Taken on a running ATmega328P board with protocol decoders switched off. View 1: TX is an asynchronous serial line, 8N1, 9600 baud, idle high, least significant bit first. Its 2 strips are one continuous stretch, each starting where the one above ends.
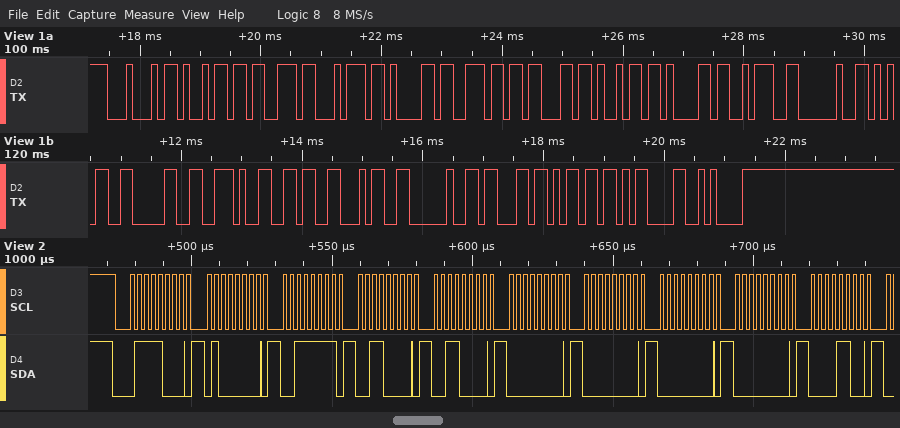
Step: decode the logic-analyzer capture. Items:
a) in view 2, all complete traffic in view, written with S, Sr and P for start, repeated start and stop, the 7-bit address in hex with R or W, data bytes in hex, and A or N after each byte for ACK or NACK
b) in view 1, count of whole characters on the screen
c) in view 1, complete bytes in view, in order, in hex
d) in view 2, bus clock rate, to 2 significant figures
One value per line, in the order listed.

S 3CW A 40 A 3F A 30 A 30 A 00 A 00 A 00 A 00 A 0C A
21
44 69 73 74 61 6E 63 69 61 3A 20 35 30 2E 36 34 20 63 6D 0D 0A
400 kHz
